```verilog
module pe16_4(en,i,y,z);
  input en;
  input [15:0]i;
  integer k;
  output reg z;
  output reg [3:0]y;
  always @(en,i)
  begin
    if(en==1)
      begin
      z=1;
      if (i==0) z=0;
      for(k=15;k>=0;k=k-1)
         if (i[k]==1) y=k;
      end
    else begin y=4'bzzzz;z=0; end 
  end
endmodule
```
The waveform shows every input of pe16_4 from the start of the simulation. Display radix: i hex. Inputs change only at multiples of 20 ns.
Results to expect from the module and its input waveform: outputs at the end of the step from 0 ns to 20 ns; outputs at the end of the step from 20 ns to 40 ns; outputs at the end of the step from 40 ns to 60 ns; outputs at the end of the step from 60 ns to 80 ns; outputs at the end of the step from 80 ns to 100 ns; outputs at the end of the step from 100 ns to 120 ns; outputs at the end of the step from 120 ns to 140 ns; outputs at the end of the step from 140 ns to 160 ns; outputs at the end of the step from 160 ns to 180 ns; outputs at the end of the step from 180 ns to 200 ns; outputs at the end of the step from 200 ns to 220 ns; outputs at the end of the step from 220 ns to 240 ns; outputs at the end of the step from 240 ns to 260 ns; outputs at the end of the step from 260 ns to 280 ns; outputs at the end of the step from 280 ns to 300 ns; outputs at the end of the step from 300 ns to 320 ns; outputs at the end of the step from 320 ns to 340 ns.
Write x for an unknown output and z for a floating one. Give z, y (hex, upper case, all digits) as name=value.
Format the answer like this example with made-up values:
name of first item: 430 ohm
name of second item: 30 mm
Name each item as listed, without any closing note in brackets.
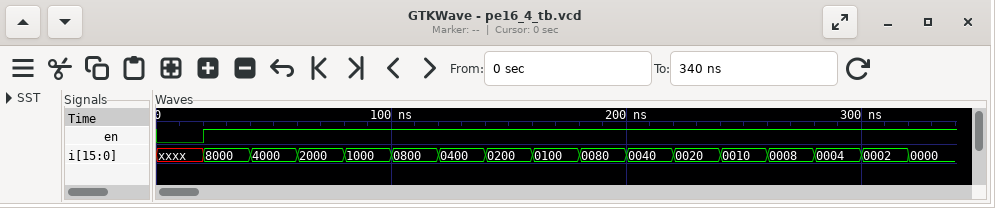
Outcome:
outputs at the end of the step from 0 ns to 20 ns: z=0, y=z
outputs at the end of the step from 20 ns to 40 ns: z=1, y=F
outputs at the end of the step from 40 ns to 60 ns: z=1, y=E
outputs at the end of the step from 60 ns to 80 ns: z=1, y=D
outputs at the end of the step from 80 ns to 100 ns: z=1, y=C
outputs at the end of the step from 100 ns to 120 ns: z=1, y=B
outputs at the end of the step from 120 ns to 140 ns: z=1, y=A
outputs at the end of the step from 140 ns to 160 ns: z=1, y=9
outputs at the end of the step from 160 ns to 180 ns: z=1, y=8
outputs at the end of the step from 180 ns to 200 ns: z=1, y=7
outputs at the end of the step from 200 ns to 220 ns: z=1, y=6
outputs at the end of the step from 220 ns to 240 ns: z=1, y=5
outputs at the end of the step from 240 ns to 260 ns: z=1, y=4
outputs at the end of the step from 260 ns to 280 ns: z=1, y=3
outputs at the end of the step from 280 ns to 300 ns: z=1, y=2
outputs at the end of the step from 300 ns to 320 ns: z=1, y=1
outputs at the end of the step from 320 ns to 340 ns: z=0, y=1
